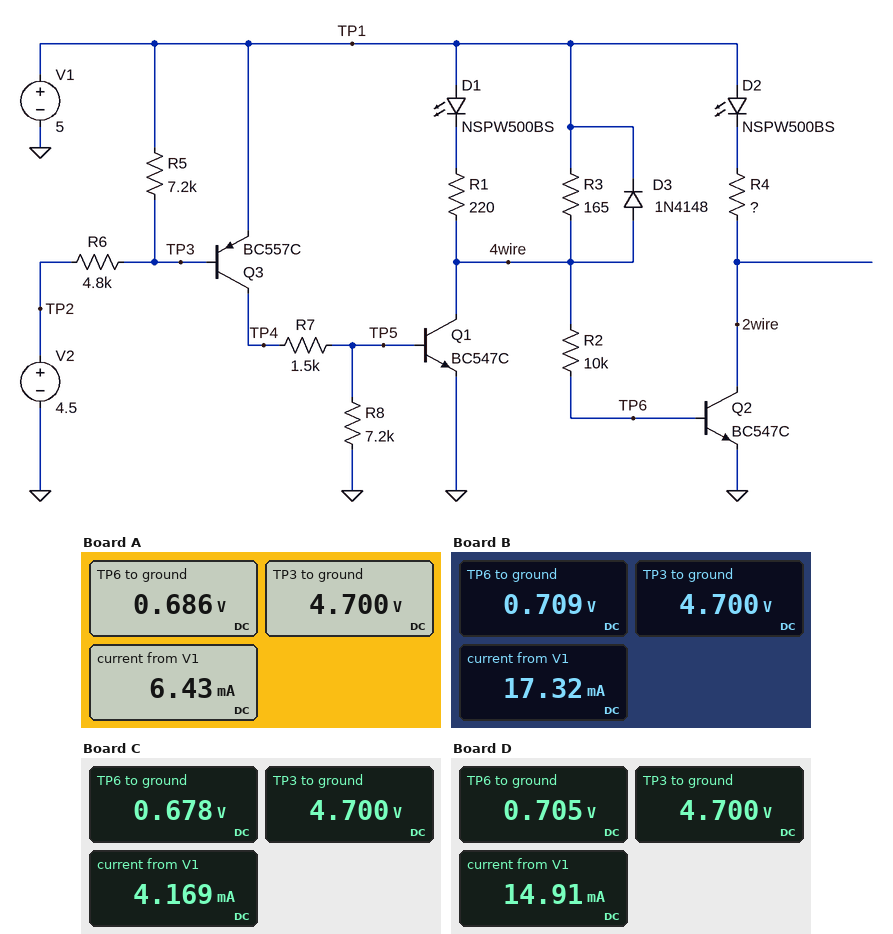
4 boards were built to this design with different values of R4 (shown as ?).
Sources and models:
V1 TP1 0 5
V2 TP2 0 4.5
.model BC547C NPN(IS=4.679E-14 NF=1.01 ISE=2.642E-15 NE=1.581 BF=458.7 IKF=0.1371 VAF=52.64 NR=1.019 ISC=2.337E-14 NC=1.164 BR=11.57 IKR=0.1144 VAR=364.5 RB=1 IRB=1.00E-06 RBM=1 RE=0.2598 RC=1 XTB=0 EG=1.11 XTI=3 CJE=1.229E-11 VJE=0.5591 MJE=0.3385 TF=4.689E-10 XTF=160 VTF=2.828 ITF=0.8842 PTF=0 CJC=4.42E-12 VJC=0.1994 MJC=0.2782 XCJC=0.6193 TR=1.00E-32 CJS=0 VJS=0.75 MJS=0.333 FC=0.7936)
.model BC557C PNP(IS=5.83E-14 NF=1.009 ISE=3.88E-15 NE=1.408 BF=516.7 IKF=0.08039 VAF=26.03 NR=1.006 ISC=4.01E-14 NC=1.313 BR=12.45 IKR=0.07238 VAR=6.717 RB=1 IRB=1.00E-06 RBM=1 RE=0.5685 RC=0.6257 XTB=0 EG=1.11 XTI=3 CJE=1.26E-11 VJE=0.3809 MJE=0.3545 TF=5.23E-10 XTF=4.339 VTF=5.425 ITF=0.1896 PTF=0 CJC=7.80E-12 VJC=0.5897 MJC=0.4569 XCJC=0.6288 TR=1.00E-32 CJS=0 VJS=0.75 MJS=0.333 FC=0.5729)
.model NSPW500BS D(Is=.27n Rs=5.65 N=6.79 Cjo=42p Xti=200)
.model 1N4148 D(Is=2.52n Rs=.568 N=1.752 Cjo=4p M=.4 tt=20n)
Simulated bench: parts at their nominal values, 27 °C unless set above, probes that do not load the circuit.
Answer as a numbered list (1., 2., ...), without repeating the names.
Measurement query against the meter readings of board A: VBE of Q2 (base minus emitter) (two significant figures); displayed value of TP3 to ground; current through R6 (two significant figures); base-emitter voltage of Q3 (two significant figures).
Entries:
1. 690 mV
2. 4.700 V
3. 42 µA
4. -300 mV
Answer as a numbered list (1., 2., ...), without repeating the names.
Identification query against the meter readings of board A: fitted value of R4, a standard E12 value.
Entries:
1. 330 Ω
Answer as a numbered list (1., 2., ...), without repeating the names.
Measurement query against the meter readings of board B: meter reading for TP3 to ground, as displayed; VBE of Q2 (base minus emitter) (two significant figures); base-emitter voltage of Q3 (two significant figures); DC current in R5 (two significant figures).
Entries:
1. 4.700 V
2. 710 mV
3. -300 mV
4. 42 µA
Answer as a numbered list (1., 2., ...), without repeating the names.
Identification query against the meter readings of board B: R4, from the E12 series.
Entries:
1. 100 Ω
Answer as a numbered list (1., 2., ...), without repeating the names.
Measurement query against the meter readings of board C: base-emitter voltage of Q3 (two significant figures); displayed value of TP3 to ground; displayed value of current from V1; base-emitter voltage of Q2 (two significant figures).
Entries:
1. -300 mV
2. 4.700 V
3. 4.169 mA
4. 680 mV
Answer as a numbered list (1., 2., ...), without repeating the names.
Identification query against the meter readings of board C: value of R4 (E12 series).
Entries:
1. 560 Ω
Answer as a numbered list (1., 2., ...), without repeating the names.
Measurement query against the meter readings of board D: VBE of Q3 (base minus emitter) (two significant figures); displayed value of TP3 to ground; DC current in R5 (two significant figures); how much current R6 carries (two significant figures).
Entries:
1. -300 mV
2. 4.700 V
3. 42 µA
4. 42 µA
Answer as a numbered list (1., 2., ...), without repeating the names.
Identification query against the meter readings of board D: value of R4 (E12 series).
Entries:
1. 120 Ω
